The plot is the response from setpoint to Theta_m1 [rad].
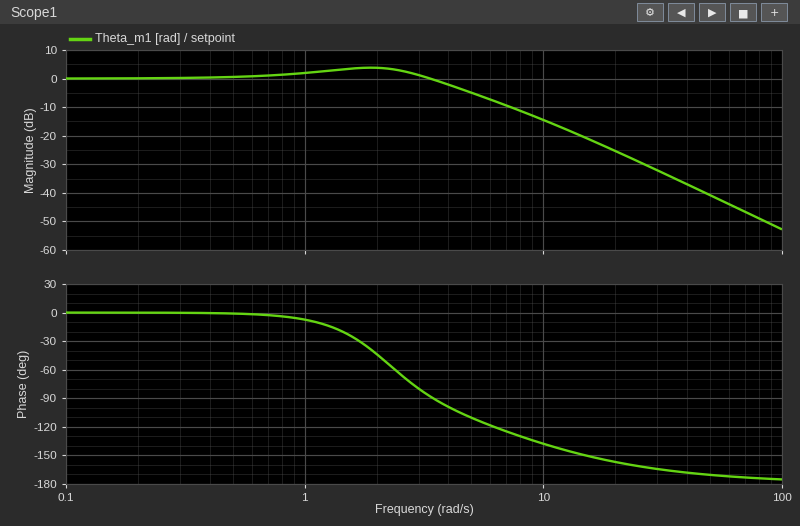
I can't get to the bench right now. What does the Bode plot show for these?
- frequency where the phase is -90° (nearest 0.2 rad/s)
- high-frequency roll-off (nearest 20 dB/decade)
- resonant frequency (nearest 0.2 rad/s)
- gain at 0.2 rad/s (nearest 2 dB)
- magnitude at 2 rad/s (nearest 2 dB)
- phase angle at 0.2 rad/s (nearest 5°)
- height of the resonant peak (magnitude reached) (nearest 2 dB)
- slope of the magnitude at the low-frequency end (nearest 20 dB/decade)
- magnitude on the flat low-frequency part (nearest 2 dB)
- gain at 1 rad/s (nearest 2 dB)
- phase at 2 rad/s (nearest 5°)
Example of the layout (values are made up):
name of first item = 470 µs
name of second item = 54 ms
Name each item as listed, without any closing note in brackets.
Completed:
frequency where the phase is -90° = 3.4 rad/s
high-frequency roll-off = -40 dB/decade
resonant frequency = 1.8 rad/s
gain at 0.2 rad/s = 0 dB
magnitude at 2 rad/s = 4 dB
phase angle at 0.2 rad/s = 0°
height of the resonant peak (magnitude reached) = 4 dB
slope of the magnitude at the low-frequency end = 0 dB/decade
magnitude on the flat low-frequency part = 0 dB
gain at 1 rad/s = 2 dB
phase at 2 rad/s = -45°
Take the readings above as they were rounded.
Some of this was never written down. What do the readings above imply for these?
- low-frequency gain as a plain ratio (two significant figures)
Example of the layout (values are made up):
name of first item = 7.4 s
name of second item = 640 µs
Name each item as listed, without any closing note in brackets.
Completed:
low-frequency gain as a plain ratio = 1.0
